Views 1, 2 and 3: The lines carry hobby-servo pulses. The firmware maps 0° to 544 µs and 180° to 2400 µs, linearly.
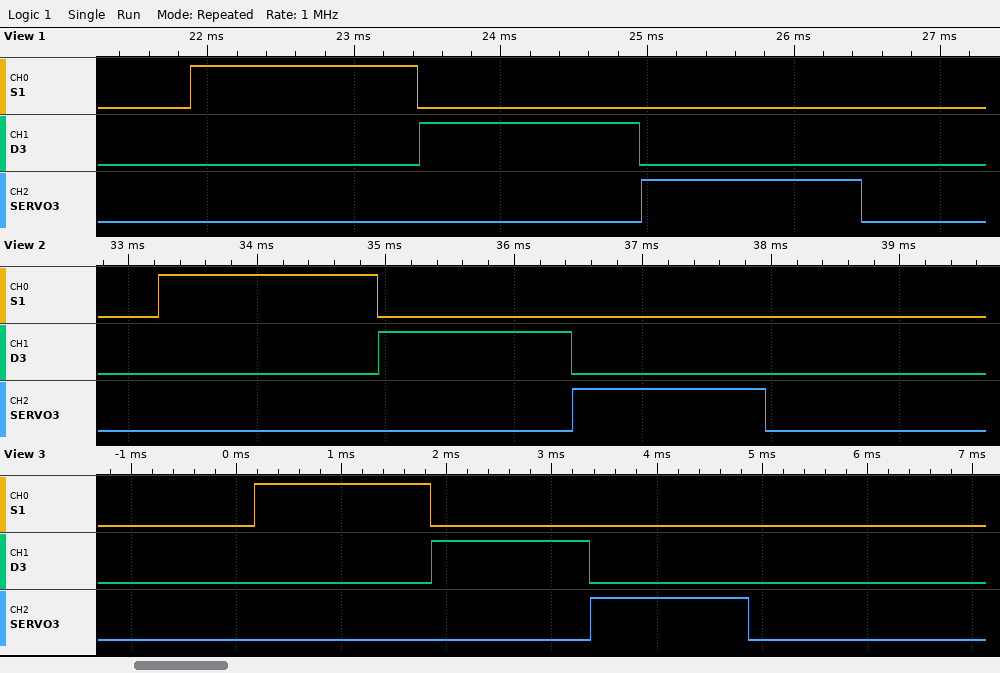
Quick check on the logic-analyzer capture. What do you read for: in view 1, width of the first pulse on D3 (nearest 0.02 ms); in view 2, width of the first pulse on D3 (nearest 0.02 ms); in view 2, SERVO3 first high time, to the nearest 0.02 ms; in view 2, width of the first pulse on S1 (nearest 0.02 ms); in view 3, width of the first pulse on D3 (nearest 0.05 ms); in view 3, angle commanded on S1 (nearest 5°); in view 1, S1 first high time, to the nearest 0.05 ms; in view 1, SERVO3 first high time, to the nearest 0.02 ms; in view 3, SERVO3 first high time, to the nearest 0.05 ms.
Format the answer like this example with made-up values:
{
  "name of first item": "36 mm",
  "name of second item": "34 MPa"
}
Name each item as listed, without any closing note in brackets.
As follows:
{
  "in view 1, width of the first pulse on D3": "1.50 ms",
  "in view 2, width of the first pulse on D3": "1.50 ms",
  "in view 2, SERVO3 first high time, to the nearest 0.02 ms": "1.50 ms",
  "in view 2, width of the first pulse on S1": "1.70 ms",
  "in view 3, width of the first pulse on D3": "1.50 ms",
  "in view 3, angle commanded on S1": "110°",
  "in view 1, S1 first high time, to the nearest 0.05 ms": "1.55 ms",
  "in view 1, SERVO3 first high time, to the nearest 0.02 ms": "1.50 ms",
  "in view 3, SERVO3 first high time, to the nearest 0.05 ms": "1.50 ms"
}
